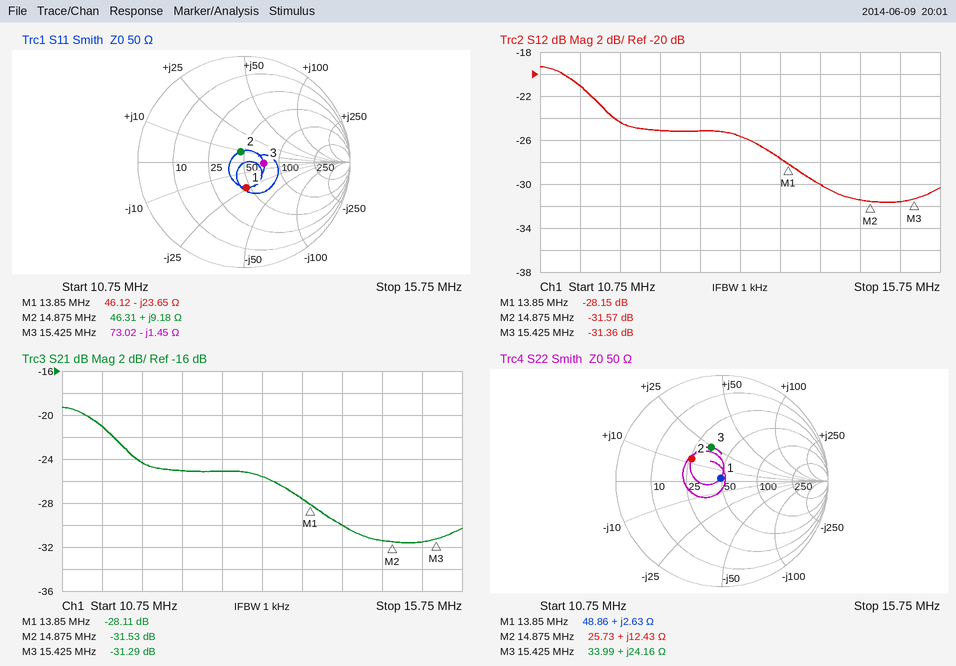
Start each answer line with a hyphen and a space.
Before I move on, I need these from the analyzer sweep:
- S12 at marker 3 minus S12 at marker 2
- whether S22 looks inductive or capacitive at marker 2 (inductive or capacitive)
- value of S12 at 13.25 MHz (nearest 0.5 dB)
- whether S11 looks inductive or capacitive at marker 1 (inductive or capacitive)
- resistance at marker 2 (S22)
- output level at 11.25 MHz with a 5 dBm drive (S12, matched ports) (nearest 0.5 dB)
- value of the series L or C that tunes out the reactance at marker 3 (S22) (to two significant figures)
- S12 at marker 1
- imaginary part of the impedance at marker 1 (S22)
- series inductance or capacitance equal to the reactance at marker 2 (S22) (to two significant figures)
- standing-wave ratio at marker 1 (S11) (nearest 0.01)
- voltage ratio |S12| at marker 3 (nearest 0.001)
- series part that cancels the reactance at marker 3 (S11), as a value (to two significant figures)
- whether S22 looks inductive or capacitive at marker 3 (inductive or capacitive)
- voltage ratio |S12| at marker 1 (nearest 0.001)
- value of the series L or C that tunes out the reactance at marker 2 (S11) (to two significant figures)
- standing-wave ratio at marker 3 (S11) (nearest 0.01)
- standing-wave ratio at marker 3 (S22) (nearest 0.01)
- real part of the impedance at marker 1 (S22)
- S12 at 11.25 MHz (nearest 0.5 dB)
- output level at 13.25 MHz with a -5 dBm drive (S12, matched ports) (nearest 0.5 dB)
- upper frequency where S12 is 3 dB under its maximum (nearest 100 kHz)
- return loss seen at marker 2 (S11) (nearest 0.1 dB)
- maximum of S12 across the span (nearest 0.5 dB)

- 0.21 dB
- inductive
- -25.5 dB
- capacitive
- 25.73 Ω
- -16.0 dBm
- 430 pF
- -28.15 dB
- +2.63 Ω
- 130 nH
- 1.64
- 0.027
- 15 nH
- inductive
- 0.039
- 1.2 nF
- 1.46
- 1.99
- 48.86 Ω
- -21.0 dB
- -30.5 dBm
- 11.4 MHz
- 19.8 dB
- -19.5 dB
